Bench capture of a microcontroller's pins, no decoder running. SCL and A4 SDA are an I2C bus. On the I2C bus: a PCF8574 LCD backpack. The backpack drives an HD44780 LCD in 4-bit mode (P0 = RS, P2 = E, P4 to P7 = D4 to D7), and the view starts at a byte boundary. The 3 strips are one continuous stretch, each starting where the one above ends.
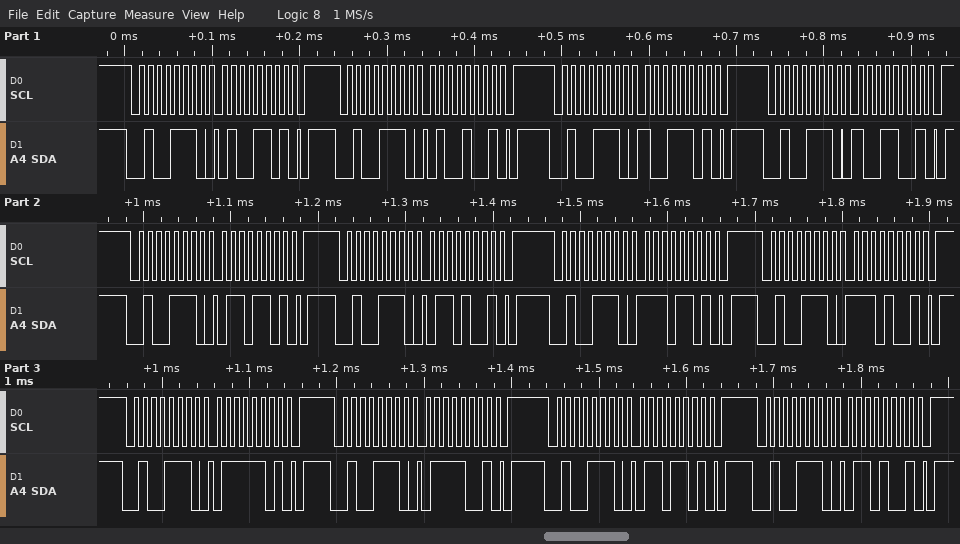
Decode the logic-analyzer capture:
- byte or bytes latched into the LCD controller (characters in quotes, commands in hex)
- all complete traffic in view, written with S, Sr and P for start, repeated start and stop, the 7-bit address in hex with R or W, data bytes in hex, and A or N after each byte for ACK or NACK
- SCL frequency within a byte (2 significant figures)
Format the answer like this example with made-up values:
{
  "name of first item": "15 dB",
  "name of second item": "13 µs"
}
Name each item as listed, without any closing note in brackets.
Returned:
{
  "byte or bytes latched into the LCD controller": "'I' 'n' 'v'",
  "all complete traffic in view, written with S, Sr and P for start, repeated start and stop, the 7-bit address in hex with R or W, data bytes in hex, and A or N after each byte for ACK or NACK": "S 27W A 4D A P S 27W A 49 A P S 27W A 9D A P S 27W A 99 A P S 27W A 6D A P S 27W A 69 A P S 27W A ED A P S 27W A E9 A P S 27W A 7D A P S 27W A 79 A P S 27W A 6D A P S 27W A 69 A P",
  "SCL frequency within a byte": "100 kHz"
}
